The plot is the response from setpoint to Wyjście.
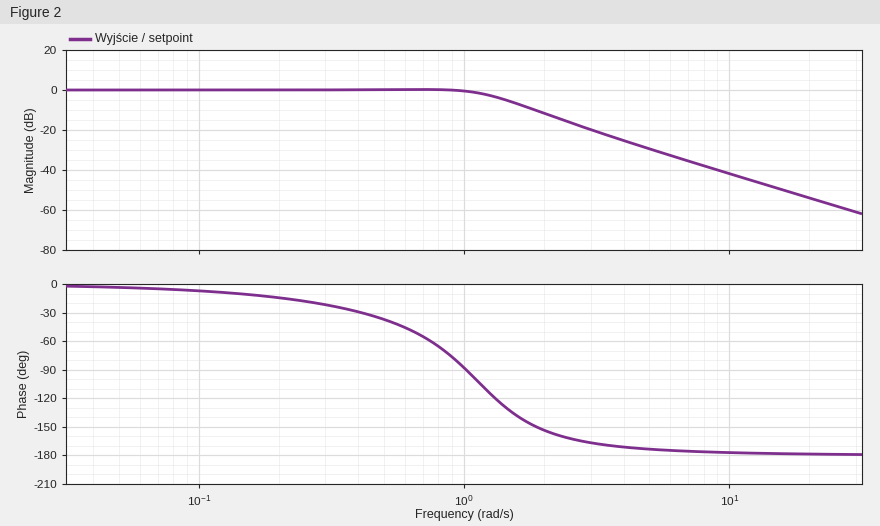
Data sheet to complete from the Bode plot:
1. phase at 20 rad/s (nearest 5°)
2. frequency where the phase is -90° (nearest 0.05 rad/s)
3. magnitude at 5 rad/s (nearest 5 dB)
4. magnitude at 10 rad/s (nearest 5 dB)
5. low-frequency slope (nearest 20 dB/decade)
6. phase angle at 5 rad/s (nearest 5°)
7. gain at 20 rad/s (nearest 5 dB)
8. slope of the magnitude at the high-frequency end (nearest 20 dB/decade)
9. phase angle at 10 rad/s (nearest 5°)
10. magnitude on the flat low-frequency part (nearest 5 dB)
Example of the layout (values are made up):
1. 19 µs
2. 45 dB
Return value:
1. -180°
2. 1.00 rad/s
3. -30 dB
4. -40 dB
5. 0 dB/decade
6. -175°
7. -55 dB
8. -40 dB/decade
9. -175°
10. 0 dB
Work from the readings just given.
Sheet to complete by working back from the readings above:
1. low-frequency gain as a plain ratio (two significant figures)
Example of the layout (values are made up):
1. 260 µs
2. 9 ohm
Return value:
1. 1.0
